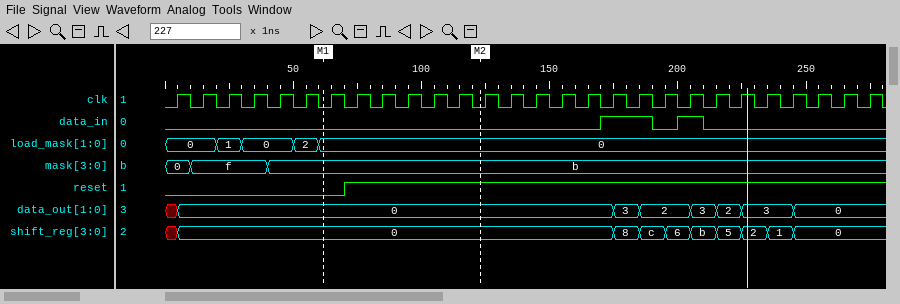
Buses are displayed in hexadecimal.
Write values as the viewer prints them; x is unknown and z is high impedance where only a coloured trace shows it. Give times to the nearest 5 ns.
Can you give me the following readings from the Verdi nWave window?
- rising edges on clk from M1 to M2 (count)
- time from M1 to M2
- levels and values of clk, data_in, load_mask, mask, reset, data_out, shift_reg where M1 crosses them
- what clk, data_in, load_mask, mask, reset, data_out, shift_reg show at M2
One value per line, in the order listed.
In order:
6
60 ns
clk=0, data_in=0, load_mask=0, mask=b, reset=0, data_out=0, shift_reg=0
clk=0, data_in=0, load_mask=0, mask=b, reset=1, data_out=0, shift_reg=0
